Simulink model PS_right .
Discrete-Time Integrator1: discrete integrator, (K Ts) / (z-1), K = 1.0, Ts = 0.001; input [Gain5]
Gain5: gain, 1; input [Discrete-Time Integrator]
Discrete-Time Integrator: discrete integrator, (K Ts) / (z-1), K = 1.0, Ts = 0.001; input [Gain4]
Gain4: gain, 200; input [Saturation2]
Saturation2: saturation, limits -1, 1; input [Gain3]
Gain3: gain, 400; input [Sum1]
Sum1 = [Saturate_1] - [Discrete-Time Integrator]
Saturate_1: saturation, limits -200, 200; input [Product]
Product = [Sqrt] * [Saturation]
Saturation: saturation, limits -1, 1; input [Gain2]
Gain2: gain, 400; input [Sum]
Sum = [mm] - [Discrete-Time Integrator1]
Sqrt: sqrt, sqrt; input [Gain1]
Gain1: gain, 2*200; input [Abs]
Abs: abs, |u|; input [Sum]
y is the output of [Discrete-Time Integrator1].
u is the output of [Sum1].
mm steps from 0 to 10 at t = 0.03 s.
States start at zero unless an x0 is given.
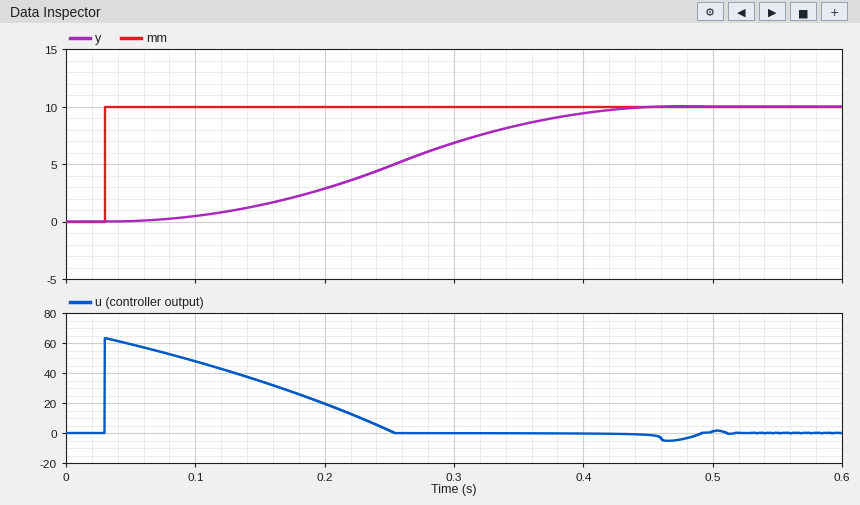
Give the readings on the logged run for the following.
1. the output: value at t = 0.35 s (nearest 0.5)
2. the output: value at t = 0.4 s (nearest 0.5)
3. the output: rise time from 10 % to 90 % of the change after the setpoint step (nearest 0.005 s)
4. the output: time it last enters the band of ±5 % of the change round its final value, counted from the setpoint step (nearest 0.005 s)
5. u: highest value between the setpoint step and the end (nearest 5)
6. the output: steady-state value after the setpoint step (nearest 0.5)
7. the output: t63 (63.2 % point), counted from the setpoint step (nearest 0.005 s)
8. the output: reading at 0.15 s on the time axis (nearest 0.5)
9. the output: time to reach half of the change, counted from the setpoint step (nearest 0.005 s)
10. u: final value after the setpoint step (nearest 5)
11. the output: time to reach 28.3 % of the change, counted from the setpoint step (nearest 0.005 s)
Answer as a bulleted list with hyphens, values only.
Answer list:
- 8.5
- 9.5
- 0.245 s
- 0.375 s
- 65
- 10.0
- 0.255 s
- 1.5
- 0.225 s
- 0
- 0.170 s
